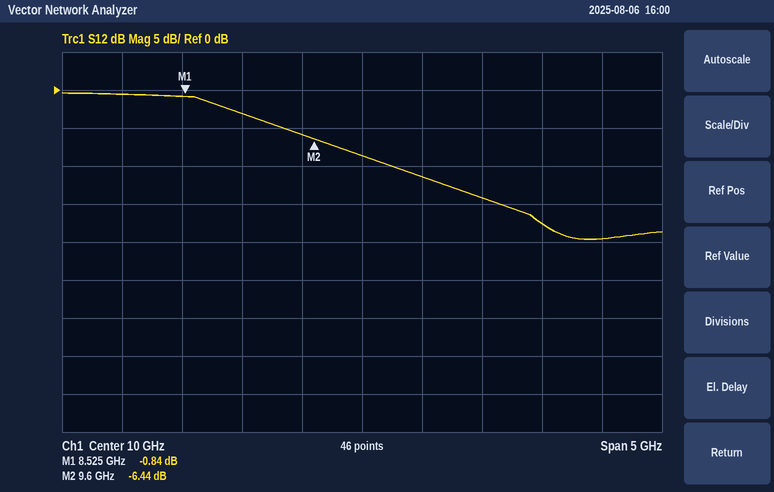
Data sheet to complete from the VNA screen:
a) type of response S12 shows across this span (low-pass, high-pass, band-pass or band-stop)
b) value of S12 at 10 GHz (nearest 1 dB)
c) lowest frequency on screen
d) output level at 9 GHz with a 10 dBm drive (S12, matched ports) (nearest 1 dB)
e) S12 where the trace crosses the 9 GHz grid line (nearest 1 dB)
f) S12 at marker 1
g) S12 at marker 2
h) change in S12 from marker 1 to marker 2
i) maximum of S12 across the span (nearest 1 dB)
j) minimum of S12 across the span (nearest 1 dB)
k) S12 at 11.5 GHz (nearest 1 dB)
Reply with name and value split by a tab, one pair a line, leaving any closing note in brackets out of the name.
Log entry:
type of response S12 shows across this span	low-pass
value of S12 at 10 GHz	-9 dB
lowest frequency on screen	7.5 GHz
output level at 9 GHz with a 10 dBm drive (S12, matched ports)	7 dBm
S12 where the trace crosses the 9 GHz grid line	-3 dB
S12 at marker 1	-0.84 dB
S12 at marker 2	-6.44 dB
change in S12 from marker 1 to marker 2	-5.60 dB
maximum of S12 across the span	0 dB
minimum of S12 across the span	-20 dB
S12 at 11.5 GHz	-18 dB
